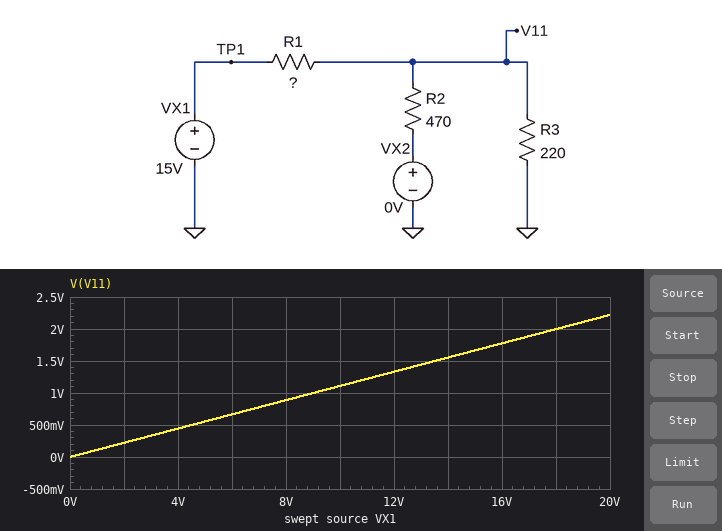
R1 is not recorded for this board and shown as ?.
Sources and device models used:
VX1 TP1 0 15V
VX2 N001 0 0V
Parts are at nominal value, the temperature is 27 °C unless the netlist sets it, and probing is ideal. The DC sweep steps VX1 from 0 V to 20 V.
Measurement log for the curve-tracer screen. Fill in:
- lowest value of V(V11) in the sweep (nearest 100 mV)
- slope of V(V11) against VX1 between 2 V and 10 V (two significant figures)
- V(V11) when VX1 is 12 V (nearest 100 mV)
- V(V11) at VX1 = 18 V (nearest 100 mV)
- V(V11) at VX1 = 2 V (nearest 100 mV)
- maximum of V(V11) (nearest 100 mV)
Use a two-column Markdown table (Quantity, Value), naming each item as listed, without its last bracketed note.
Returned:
| Quantity | Value |
|---|---|
| lowest value of V(V11) in the sweep | 0 V |
| slope of V(V11) against VX1 between 2 V and 10 V | 0.11 V/V |
| V(V11) when VX1 is 12 V | 1.3 V |
| V(V11) at VX1 = 18 V | 2.0 V |
| V(V11) at VX1 = 2 V | 200 mV |
| maximum of V(V11) | 2.2 V |
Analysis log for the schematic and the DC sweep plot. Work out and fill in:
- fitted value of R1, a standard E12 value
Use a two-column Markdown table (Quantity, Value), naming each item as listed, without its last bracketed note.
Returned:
| Quantity | Value |
|---|---|
| fitted value of R1, a standard E12 value | 1.2 kΩ |
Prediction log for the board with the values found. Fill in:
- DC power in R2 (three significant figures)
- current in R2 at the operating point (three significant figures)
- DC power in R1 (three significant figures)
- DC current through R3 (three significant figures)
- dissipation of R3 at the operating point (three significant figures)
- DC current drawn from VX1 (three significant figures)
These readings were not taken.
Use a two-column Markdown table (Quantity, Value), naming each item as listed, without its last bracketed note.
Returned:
| Quantity | Value |
|---|---|
| DC power in R2 | 5.90 mW |
| current in R2 at the operating point | 3.54 mA |
| DC power in R1 | 148 mW |
| DC current through R3 | 7.57 mA |
| dissipation of R3 at the operating point | 12.6 mW |
| DC current drawn from VX1 | 11.1 mA |
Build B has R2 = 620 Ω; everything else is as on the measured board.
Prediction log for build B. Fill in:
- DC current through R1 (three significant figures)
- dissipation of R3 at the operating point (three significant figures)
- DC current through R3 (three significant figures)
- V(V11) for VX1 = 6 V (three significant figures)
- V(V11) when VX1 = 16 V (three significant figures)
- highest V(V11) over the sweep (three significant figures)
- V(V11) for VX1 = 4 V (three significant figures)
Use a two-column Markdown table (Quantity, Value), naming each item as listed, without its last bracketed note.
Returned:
| Quantity | Value |
|---|---|
| DC current through R1 | 11.0 mA |
| dissipation of R3 at the operating point | 14.5 mW |
| DC current through R3 | 8.13 mA |
| V(V11) for VX1 = 6 V | 715 mV |
| V(V11) when VX1 = 16 V | 1.91 V |
| highest V(V11) over the sweep | 2.38 V |
| V(V11) for VX1 = 4 V | 477 mV |
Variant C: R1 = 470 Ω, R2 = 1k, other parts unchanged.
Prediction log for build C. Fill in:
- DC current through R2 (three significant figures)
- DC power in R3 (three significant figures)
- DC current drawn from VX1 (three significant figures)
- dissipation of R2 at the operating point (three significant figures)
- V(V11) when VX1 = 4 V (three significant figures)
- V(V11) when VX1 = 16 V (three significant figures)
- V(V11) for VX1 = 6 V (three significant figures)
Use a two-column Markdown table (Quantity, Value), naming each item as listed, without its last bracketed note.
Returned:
| Quantity | Value |
|---|---|
| DC current through R2 | 4.16 mA |
| DC power in R3 | 78.6 mW |
| DC current drawn from VX1 | 23.1 mA |
| dissipation of R2 at the operating point | 17.3 mW |
| V(V11) when VX1 = 4 V | 1.11 V |
| V(V11) when VX1 = 16 V | 4.44 V |
| V(V11) for VX1 = 6 V | 1.66 V |
